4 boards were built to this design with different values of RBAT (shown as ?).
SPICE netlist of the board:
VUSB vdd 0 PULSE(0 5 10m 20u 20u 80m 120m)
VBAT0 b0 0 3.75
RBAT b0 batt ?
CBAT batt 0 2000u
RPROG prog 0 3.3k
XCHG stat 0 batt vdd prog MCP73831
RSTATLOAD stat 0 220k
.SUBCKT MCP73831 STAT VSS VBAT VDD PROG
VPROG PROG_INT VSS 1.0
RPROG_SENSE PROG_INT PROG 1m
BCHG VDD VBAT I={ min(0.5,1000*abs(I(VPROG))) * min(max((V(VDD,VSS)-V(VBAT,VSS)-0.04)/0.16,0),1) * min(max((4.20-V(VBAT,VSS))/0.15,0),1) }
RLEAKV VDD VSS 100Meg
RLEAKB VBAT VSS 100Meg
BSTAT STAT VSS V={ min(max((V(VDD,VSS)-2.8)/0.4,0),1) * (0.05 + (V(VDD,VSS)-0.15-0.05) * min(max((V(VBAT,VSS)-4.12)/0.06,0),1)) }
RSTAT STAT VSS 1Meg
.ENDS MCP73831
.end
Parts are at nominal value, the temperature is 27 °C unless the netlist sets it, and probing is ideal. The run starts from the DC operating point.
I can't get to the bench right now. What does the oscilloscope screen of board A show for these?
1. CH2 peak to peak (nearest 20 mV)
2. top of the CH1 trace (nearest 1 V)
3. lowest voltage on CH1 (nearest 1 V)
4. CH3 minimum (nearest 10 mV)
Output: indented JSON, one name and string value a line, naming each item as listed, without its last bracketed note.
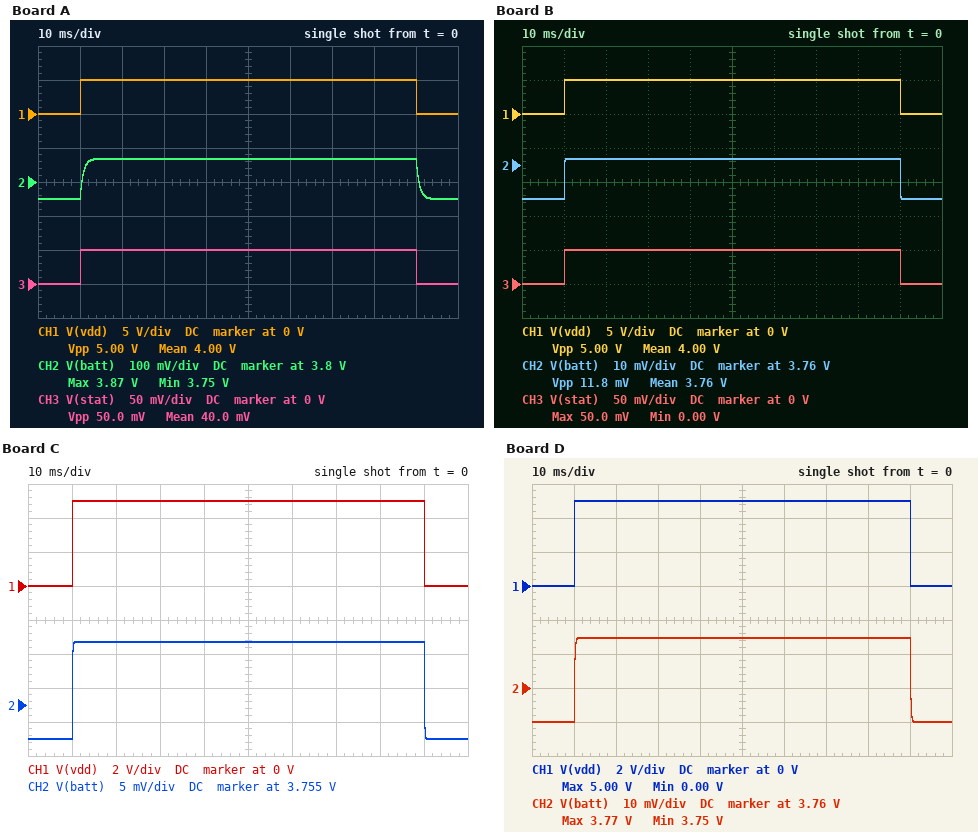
{
  "CH2 peak to peak": "120 mV",
  "top of the CH1 trace": "5 V",
  "lowest voltage on CH1": "0 V",
  "CH3 minimum": "0 V"
}
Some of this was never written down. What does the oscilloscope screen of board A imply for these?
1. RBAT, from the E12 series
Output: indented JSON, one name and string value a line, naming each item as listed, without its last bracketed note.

{
  "RBAT, from the E12 series": "0.39 Ω"
}
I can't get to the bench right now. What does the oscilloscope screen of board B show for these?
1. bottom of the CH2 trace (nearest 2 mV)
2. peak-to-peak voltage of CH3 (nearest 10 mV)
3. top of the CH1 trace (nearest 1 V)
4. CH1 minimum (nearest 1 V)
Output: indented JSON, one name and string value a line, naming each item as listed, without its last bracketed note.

{
  "bottom of the CH2 trace": "3.750 V",
  "peak-to-peak voltage of CH3": "50 mV",
  "top of the CH1 trace": "5 V",
  "CH1 minimum": "0 V"
}
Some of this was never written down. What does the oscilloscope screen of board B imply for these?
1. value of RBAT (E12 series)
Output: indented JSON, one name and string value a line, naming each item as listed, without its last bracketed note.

{
  "value of RBAT": "0.039 Ω"
}
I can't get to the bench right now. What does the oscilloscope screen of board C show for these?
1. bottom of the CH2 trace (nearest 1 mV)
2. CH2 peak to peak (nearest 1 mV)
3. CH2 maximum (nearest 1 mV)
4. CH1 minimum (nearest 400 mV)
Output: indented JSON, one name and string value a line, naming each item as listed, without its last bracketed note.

{
  "bottom of the CH2 trace": "3.750 V",
  "CH2 peak to peak": "14 mV",
  "CH2 maximum": "3.764 V",
  "CH1 minimum": "0 V"
}
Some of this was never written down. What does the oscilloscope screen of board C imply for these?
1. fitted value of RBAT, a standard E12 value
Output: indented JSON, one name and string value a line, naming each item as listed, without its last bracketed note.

{
  "fitted value of RBAT, a standard E12 value": "0.047 Ω"
}
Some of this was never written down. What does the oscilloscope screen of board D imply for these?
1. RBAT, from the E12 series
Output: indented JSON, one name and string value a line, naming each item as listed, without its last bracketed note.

{
  "RBAT, from the E12 series": "0.082 Ω"
}
